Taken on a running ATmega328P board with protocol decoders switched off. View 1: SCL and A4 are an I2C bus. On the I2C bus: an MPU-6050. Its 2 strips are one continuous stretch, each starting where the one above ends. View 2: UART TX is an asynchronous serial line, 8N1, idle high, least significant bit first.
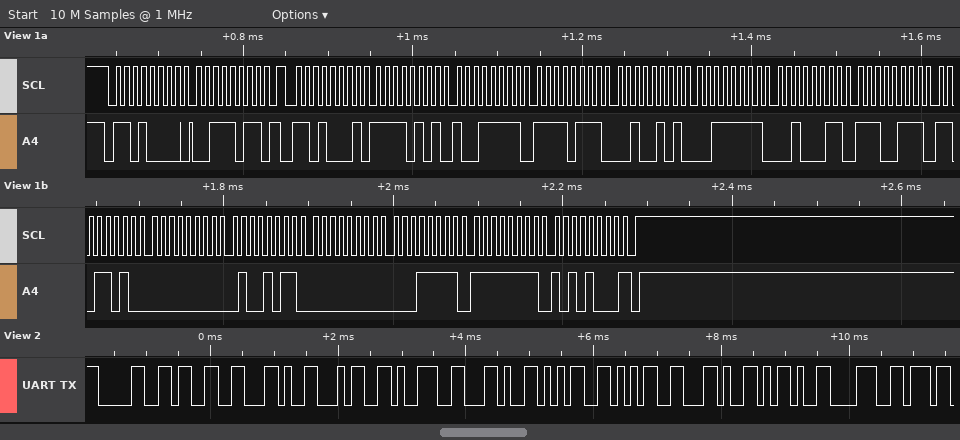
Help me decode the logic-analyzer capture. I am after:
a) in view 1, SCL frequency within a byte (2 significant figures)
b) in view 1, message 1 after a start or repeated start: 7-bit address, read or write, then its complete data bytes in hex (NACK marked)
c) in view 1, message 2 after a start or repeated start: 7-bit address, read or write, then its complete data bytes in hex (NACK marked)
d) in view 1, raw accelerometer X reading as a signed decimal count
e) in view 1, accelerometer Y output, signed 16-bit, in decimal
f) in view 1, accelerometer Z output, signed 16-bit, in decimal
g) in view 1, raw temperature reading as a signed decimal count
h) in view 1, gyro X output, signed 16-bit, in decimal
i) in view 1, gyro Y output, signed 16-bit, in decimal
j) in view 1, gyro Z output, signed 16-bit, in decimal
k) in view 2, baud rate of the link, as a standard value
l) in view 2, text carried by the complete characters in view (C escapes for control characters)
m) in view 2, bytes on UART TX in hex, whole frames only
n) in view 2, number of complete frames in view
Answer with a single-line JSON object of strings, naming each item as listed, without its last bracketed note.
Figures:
{"in view 1, SCL frequency within a byte": "100 kHz", "in view 1, message 1 after a start or repeated start: 7-bit address, read or write, then its complete data bytes in hex": "0x68 write: 3B", "in view 1, message 2 after a start or repeated start: 7-bit address, read or write, then its complete data bytes in hex": "0x68 read: F5 9F F7 25 3F 23 E7 DA 00 4B 00 1F FF A8 NACK", "in view 1, raw accelerometer X reading as a signed decimal count": "-2657", "in view 1, accelerometer Y output, signed 16-bit, in decimal": "-2267", "in view 1, accelerometer Z output, signed 16-bit, in decimal": "16163", "in view 1, raw temperature reading as a signed decimal count": "-6182", "in view 1, gyro X output, signed 16-bit, in decimal": "75", "in view 1, gyro Y output, signed 16-bit, in decimal": "31", "in view 1, gyro Z output, signed 16-bit, in decimal": "-88", "in view 2, baud rate of the link, as a standard value": "9600 baud", "in view 2, text carried by the complete characters in view": "\"03,49,55,-8\"", "in view 2, bytes on UART TX in hex, whole frames only": "30 33 2C 34 39 2C 35 35 2C 2D 38", "in view 2, number of complete frames in view": "11"}
